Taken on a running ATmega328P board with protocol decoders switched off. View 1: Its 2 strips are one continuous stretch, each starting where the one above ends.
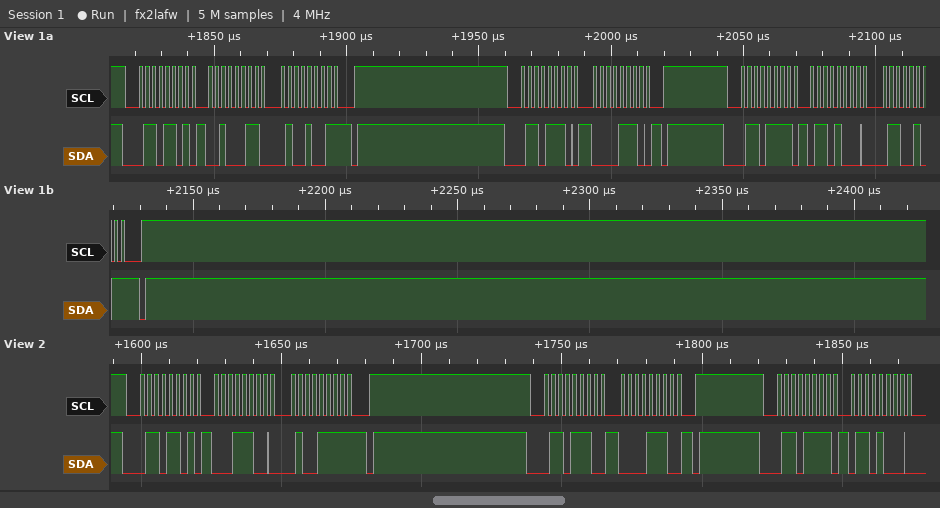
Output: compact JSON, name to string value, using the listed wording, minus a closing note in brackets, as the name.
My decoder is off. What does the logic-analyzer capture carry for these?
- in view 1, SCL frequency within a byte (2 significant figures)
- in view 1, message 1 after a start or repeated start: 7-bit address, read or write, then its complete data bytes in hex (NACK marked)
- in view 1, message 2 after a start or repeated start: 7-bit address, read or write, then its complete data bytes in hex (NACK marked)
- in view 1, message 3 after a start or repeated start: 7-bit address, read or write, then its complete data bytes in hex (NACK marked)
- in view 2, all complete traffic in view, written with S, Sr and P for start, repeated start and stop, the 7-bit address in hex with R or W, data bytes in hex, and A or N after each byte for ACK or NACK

{"in view 1, SCL frequency within a byte": "400 kHz", "in view 1, message 1 after a start or repeated start: 7-bit address, read or write, then its complete data bytes in hex": "0x36 read: 23 49 NACK", "in view 1, message 2 after a start or repeated start: 7-bit address, read or write, then its complete data bytes in hex": "0x37 write: 0E", "in view 1, message 3 after a start or repeated start: 7-bit address, read or write, then its complete data bytes in hex": "0x37 read: 68 65 NACK", "in view 2, all complete traffic in view, written with S, Sr and P for start, repeated start and stop, the 7-bit address in hex with R or W, data bytes in hex, and A or N after each byte for ACK or NACK": "S 36R A 1C A 4F N P S 37W A 0E A P S 37R A 68 A"}
